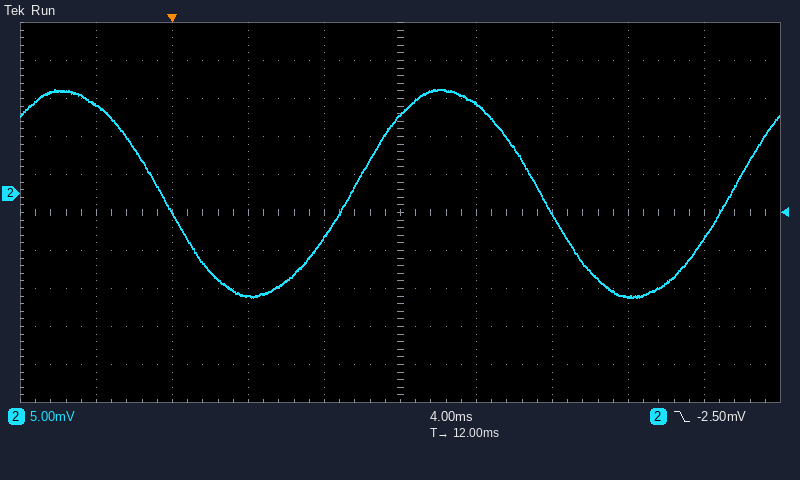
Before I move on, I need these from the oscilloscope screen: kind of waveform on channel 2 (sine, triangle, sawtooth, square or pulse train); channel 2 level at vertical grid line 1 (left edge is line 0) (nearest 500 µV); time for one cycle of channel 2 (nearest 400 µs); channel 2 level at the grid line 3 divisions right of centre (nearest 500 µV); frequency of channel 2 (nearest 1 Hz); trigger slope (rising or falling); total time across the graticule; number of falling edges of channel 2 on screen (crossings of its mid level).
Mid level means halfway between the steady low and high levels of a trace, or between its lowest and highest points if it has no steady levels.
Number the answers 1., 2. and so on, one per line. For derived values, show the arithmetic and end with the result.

1. sine
2. 11.5 mV
3. 20.0 ms
4. -13.5 mV
5. 1 / 20.0 ms ≈ 50 Hz
6. falling
7. 40 ms
8. 2
